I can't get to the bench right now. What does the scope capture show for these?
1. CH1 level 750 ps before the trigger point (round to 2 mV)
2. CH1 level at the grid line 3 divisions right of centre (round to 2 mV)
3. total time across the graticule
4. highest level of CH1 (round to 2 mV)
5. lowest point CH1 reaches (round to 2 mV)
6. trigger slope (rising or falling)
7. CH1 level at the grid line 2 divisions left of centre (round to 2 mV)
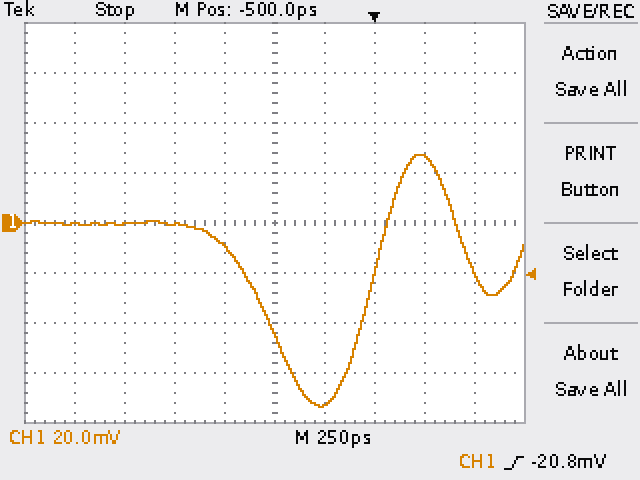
-10 mV
26 mV
2.5 ns
28 mV
-74 mV
rising
0 mV
